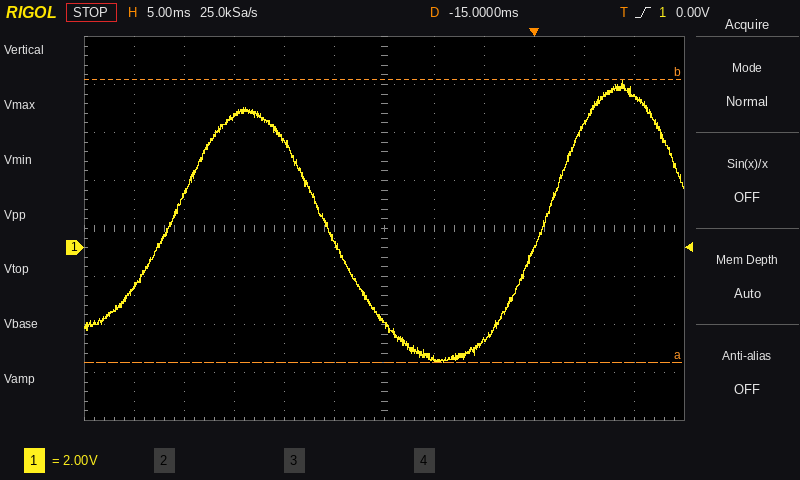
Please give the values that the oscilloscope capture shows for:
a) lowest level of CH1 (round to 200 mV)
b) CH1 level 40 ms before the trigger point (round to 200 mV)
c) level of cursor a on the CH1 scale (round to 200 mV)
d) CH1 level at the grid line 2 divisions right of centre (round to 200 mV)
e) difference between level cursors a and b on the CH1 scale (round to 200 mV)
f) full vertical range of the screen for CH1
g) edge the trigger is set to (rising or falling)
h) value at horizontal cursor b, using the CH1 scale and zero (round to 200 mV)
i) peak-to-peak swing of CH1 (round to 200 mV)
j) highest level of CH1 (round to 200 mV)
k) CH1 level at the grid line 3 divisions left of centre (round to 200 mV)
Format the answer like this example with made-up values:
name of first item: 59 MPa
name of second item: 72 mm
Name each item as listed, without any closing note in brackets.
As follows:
lowest level of CH1: -4.8 V
CH1 level 40 ms before the trigger point: -1.6 V
level of cursor a on the CH1 scale: -4.8 V
CH1 level at the grid line 2 divisions right of centre: -3.8 V
difference between level cursors a and b on the CH1 scale: 11.8 V
full vertical range of the screen for CH1: 16 V
edge the trigger is set to: rising
value at horizontal cursor b, using the CH1 scale and zero: 7.0 V
peak-to-peak swing of CH1: 11.8 V
highest level of CH1: 7.0 V
CH1 level at the grid line 3 divisions left of centre: 5.4 V
